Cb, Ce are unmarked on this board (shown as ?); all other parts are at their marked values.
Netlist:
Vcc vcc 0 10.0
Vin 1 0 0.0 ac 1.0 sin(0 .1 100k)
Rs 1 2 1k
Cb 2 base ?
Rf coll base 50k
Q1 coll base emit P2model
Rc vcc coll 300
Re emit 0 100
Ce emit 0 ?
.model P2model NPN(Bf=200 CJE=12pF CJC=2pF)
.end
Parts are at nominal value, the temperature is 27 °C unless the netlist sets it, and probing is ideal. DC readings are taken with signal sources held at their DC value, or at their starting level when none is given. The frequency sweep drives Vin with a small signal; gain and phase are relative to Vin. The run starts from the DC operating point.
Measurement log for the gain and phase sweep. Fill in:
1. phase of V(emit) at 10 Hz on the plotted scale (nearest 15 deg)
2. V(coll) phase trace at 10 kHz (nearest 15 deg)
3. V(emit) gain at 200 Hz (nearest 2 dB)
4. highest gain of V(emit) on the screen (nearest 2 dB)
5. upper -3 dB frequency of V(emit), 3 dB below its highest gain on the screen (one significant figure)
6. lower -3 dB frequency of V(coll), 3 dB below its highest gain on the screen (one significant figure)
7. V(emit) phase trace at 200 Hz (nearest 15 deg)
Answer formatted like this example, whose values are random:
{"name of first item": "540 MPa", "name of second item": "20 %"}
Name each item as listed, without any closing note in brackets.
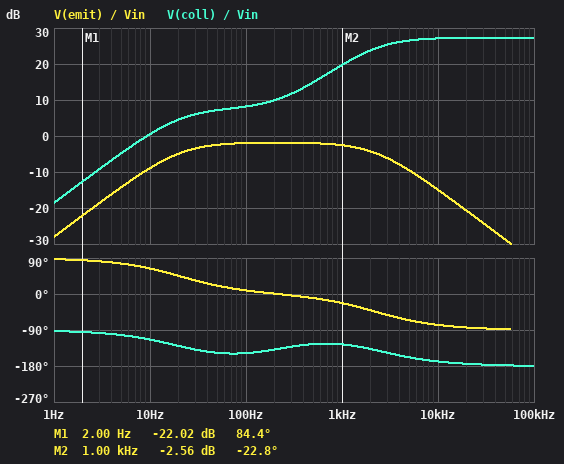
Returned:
{"phase of V(emit) at 10 Hz on the plotted scale": "60 deg", "V(coll) phase trace at 10 kHz": "-165 deg", "V(emit) gain at 200 Hz": "-2 dB", "highest gain of V(emit) on the screen": "-2 dB", "upper -3 dB frequency of V(emit), 3 dB below its highest gain on the screen": "2 kHz", "lower -3 dB frequency of V(coll), 3 dB below its highest gain on the screen": "2 kHz", "V(emit) phase trace at 200 Hz": "0 deg"}
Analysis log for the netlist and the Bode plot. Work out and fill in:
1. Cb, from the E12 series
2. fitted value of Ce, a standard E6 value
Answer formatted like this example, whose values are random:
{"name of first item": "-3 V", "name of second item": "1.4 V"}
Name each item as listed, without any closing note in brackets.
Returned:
{"Cb, from the E12 series": "820 nF", "fitted value of Ce, a standard E6 value": "6.8 µF"}
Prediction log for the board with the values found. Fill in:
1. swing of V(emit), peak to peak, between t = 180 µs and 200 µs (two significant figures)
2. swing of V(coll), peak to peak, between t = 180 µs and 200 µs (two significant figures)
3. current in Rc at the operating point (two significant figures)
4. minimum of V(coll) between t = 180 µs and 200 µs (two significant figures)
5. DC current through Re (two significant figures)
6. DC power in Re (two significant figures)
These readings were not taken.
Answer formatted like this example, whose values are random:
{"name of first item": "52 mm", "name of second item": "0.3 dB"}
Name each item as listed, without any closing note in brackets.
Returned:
{"swing of V(emit), peak to peak, between t = 180 µs and 200 µs": "3.6 mV", "swing of V(coll), peak to peak, between t = 180 µs and 200 µs": "4.6 V", "current in Rc at the operating point": "14 mA", "minimum of V(coll) between t = 180 µs and 200 µs": "3.4 V", "DC current through Re": "14 mA", "DC power in Re": "20 mW"}
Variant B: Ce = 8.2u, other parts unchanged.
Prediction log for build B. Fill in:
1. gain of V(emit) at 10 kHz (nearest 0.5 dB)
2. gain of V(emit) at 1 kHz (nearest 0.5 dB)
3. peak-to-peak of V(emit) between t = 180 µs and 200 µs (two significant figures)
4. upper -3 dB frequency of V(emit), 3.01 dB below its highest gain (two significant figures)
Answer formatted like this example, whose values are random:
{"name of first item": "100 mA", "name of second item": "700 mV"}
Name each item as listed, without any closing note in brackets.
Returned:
{"gain of V(emit) at 10 kHz": "-16.5 dB", "gain of V(emit) at 1 kHz": "-3.0 dB", "peak-to-peak of V(emit) between t = 180 µs and 200 µs": "3.0 mV", "upper -3 dB frequency of V(emit), 3.01 dB below its highest gain": "1.9 kHz"}
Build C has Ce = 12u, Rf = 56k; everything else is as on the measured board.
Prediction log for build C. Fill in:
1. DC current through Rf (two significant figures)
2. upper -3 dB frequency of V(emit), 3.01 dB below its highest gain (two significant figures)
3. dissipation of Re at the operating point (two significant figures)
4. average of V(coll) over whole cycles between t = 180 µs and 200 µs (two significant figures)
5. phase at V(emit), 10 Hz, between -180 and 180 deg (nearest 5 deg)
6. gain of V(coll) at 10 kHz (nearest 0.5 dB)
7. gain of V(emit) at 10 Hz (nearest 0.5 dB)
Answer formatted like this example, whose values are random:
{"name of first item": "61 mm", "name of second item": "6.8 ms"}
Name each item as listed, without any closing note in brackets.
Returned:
{"DC current through Rf": "67 µA", "upper -3 dB frequency of V(emit), 3.01 dB below its highest gain": "1.4 kHz", "dissipation of Re at the operating point": "18 mW", "average of V(coll) over whole cycles between t = 180 µs and 200 µs": "5.9 V", "phase at V(emit), 10 Hz, between -180 and 180 deg": "60 deg", "gain of V(coll) at 10 kHz": "27.5 dB", "gain of V(emit) at 10 Hz": "-8.5 dB"}
